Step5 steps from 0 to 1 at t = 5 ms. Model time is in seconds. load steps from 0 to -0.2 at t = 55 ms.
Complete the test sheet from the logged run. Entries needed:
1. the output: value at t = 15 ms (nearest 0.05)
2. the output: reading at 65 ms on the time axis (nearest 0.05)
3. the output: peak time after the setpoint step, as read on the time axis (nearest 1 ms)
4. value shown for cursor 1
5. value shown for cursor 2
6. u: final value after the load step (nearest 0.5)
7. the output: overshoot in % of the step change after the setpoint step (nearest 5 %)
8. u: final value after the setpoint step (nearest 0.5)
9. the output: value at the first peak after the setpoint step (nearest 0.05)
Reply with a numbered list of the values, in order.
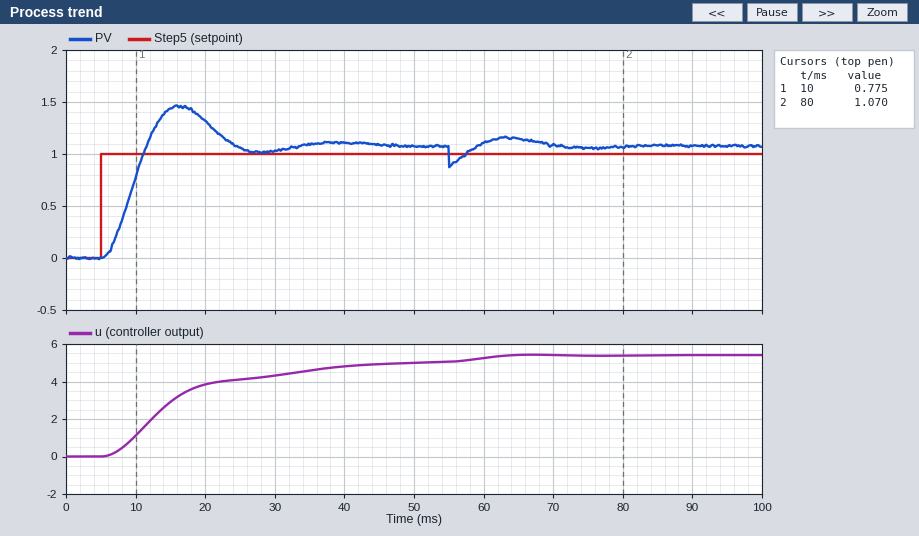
1. 1.45
2. 1.15
3. 16 ms
4. 0.775
5. 1.070
6. 5.5
7. 35 %
8. 5.0
9. 1.45
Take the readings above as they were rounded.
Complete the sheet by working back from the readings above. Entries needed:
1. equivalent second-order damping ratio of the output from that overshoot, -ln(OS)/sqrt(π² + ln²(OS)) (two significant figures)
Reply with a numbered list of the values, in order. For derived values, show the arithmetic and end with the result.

1. ln(0.35) = -1.050; 1.050 / sqrt(9.870 + 1.102) = 0.32
